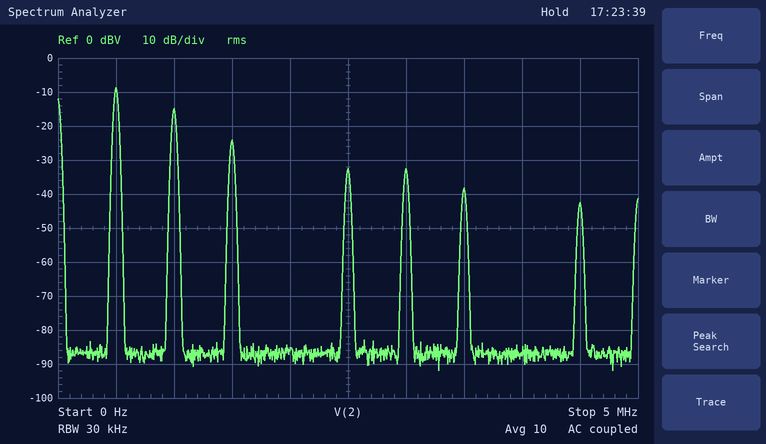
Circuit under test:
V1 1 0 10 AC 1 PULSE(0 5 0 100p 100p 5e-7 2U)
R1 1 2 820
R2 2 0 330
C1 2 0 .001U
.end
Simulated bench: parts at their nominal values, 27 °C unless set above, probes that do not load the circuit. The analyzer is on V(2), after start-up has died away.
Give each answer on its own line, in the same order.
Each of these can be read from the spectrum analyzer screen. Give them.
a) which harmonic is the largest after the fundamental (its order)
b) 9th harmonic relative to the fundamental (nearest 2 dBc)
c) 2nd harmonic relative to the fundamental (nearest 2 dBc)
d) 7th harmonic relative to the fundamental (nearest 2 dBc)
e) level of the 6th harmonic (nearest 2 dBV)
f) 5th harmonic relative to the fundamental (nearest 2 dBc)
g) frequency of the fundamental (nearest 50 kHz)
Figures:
2
-34 dBc
-6 dBc
-30 dBc
-32 dBV
-24 dBc
500 kHz
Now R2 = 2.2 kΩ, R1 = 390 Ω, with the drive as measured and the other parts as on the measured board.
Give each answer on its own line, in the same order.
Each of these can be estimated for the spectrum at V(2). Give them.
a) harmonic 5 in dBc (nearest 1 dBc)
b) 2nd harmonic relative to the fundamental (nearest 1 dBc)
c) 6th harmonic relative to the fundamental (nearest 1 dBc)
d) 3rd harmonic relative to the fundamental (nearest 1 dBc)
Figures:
-25 dBc
-7 dBc
-25 dBc
-17 dBc
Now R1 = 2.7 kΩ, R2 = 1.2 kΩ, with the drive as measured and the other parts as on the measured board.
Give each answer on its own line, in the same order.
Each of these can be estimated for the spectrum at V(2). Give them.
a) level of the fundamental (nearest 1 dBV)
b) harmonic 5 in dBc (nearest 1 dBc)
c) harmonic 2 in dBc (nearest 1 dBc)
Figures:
-15 dBV
-27 dBc
-9 dBc
